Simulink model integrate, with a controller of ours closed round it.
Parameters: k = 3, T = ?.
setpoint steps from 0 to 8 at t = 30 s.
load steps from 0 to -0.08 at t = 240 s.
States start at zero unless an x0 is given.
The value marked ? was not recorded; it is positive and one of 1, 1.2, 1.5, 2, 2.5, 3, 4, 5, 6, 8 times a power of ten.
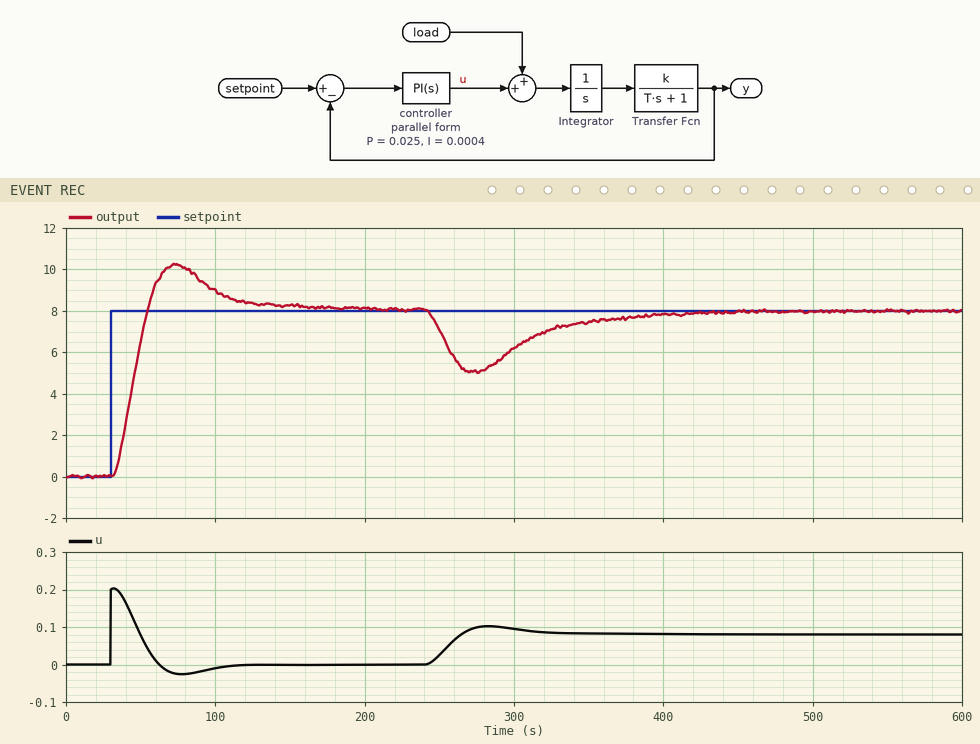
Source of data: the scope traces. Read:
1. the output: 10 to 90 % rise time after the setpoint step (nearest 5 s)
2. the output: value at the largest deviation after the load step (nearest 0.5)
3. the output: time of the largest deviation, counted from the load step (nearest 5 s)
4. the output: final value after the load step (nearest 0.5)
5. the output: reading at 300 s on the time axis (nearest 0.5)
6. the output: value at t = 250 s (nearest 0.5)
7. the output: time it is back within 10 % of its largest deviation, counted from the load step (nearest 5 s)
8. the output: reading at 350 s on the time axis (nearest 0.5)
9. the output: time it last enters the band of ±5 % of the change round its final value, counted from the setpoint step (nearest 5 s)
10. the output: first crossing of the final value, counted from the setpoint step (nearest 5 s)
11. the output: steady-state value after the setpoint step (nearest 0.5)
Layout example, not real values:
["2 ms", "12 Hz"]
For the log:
["15 s", "5.0", "35 s", "8.0", "6.0", "7.0", "140 s", "7.5", "90 s", "25 s", "8.0"]
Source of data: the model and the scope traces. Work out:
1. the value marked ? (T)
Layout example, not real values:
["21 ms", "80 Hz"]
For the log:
["8"]
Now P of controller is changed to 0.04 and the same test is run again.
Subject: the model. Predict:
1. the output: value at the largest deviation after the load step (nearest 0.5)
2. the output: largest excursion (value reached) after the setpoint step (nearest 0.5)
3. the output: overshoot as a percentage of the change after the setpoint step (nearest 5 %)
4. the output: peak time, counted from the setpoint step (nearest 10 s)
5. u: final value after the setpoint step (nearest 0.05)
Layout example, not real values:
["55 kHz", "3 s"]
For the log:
["6.0", "10.0", "25 %", "30 s", "0.00"]
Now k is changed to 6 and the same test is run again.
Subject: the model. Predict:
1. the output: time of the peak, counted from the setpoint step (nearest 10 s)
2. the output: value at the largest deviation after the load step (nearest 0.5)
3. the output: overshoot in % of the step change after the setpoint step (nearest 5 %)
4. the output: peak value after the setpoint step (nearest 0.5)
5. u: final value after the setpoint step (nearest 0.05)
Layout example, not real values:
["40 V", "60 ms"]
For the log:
["30 s", "4.5", "35 %", "11.0", "0.00"]
